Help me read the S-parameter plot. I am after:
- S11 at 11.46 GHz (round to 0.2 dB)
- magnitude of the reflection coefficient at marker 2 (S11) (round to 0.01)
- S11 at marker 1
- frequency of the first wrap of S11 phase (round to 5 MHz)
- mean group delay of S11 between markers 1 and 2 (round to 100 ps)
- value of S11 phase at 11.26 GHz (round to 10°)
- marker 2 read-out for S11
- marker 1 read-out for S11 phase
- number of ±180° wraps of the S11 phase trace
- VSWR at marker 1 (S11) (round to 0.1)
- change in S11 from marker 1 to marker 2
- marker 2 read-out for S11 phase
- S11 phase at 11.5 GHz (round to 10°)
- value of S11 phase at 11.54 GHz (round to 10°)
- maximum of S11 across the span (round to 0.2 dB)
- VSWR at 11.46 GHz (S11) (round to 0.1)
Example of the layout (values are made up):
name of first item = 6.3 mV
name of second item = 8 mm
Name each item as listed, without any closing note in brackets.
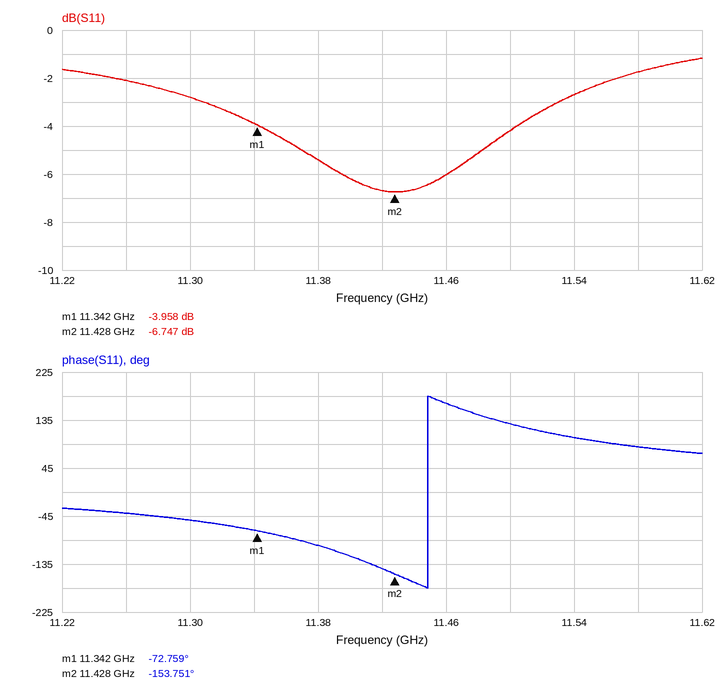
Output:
S11 at 11.46 GHz = -6.0 dB
magnitude of the reflection coefficient at marker 2 (S11) = 0.46
S11 at marker 1 = -3.958 dB
frequency of the first wrap of S11 phase = 11.450 GHz
mean group delay of S11 between markers 1 and 2 = 2.6 ns
value of S11 phase at 11.26 GHz = -40°
marker 2 read-out for S11 = -6.747 dB
marker 1 read-out for S11 phase = -72.759°
number of ±180° wraps of the S11 phase trace = 1
VSWR at marker 1 (S11) = 4.5
change in S11 from marker 1 to marker 2 = -2.789 dB
marker 2 read-out for S11 phase = -153.751°
S11 phase at 11.5 GHz = 130°
value of S11 phase at 11.54 GHz = 100°
maximum of S11 across the span = -1.2 dB
VSWR at 11.46 GHz (S11) = 3.0
